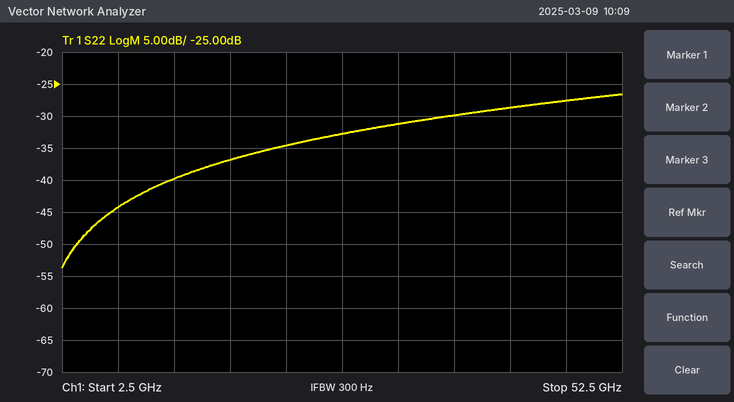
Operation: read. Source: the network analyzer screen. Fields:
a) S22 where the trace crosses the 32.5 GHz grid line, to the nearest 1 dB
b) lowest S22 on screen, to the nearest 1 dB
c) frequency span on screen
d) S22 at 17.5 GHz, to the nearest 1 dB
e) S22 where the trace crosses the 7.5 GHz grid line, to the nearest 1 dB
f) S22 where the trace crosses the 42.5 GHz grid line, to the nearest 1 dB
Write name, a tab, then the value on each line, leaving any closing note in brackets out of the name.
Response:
S22 where the trace crosses the 32.5 GHz grid line, to the nearest 1 dB	-31 dB
lowest S22 on screen, to the nearest 1 dB	-54 dB
frequency span on screen	50 GHz
S22 at 17.5 GHz, to the nearest 1 dB	-37 dB
S22 where the trace crosses the 7.5 GHz grid line, to the nearest 1 dB	-44 dB
S22 where the trace crosses the 42.5 GHz grid line, to the nearest 1 dB	-29 dB
